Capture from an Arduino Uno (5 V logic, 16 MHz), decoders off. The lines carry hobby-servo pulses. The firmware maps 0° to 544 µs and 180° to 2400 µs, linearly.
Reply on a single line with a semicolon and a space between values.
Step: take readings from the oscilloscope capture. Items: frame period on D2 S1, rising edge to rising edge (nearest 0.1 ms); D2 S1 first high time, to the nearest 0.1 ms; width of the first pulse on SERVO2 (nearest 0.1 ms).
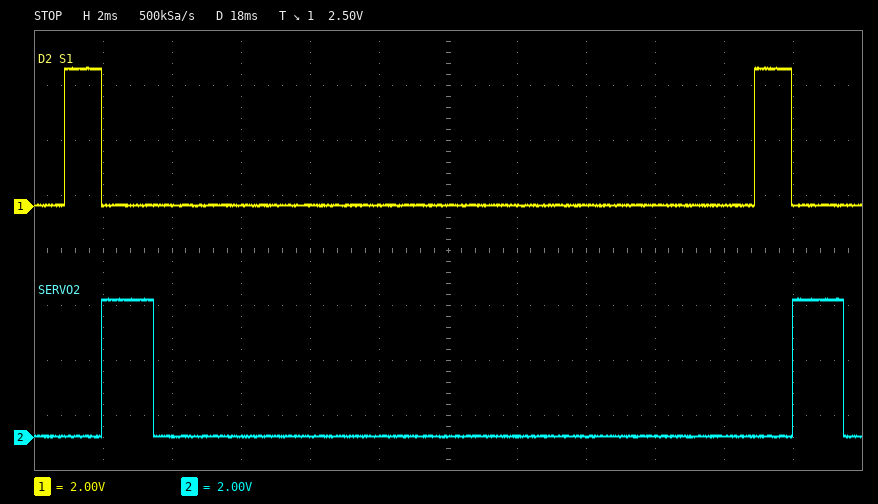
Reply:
20.0 ms; 1.1 ms; 1.5 ms
